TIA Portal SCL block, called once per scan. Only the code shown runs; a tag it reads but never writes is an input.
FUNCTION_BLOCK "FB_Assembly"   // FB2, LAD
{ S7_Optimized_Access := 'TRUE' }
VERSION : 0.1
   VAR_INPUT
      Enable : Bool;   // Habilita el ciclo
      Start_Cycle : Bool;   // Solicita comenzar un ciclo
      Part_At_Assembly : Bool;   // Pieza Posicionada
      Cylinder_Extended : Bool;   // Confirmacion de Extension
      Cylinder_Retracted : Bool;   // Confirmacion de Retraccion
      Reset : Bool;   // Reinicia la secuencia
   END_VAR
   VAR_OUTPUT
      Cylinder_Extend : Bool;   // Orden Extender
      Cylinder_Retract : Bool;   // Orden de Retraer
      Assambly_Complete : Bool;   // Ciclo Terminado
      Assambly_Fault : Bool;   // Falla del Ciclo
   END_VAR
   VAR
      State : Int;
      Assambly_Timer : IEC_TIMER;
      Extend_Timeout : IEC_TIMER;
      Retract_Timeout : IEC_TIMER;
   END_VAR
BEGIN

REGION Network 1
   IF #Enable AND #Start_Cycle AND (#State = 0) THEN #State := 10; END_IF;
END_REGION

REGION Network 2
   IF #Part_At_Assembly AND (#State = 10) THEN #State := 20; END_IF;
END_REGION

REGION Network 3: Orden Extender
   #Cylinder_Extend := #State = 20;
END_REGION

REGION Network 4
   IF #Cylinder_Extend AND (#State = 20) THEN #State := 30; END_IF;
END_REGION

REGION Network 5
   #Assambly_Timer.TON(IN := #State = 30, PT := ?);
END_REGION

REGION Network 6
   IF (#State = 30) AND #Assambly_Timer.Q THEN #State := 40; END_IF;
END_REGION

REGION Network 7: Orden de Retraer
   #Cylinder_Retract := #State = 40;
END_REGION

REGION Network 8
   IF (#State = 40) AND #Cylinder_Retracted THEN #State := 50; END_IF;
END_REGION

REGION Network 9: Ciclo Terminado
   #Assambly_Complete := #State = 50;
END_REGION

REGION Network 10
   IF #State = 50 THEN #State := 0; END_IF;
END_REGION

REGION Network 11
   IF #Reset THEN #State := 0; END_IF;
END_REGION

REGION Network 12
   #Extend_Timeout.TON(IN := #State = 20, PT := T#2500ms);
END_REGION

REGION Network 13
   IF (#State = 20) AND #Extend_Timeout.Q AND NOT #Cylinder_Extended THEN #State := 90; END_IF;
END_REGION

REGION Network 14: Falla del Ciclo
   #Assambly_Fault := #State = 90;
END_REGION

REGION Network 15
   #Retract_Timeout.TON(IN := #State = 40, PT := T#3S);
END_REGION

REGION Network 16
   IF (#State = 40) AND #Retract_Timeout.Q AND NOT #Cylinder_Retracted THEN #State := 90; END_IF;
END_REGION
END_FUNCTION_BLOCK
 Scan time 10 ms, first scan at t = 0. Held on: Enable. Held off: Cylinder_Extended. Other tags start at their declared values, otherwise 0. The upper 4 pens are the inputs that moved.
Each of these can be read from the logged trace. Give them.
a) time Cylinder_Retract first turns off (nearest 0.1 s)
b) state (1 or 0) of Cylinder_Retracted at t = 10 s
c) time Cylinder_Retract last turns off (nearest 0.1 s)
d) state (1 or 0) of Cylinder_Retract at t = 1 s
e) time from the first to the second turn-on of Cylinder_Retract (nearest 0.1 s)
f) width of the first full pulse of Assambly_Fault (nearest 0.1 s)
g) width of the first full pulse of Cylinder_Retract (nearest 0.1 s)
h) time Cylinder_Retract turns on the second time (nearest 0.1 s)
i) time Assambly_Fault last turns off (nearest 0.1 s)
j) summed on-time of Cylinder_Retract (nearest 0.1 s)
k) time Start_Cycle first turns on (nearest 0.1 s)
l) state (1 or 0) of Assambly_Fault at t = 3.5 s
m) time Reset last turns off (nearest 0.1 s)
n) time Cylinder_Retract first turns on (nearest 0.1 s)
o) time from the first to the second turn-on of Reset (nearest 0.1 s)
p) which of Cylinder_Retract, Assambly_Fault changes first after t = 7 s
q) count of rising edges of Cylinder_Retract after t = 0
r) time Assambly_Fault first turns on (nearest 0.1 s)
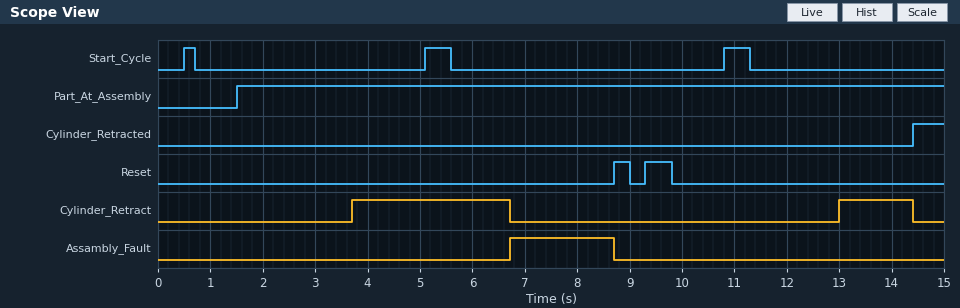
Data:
6.7 s
0
14.4 s
0
9.3 s
2.0 s
3.0 s
13.0 s
8.7 s
4.4 s
0.5 s
0
9.8 s
3.7 s
0.6 s
Assambly_Fault
2
6.7 s
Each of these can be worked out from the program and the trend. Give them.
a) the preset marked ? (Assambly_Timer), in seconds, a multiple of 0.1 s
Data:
2.2 s
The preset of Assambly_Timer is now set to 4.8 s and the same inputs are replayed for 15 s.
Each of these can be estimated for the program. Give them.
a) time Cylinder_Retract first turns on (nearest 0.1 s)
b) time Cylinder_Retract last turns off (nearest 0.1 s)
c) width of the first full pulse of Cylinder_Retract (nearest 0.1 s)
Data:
6.3 s
8.7 s
2.4 s
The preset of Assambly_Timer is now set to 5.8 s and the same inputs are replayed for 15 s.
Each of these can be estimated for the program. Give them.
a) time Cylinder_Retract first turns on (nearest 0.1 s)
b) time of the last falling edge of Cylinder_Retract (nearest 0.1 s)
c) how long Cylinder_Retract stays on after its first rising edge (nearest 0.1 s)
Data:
7.3 s
8.7 s
1.4 s
